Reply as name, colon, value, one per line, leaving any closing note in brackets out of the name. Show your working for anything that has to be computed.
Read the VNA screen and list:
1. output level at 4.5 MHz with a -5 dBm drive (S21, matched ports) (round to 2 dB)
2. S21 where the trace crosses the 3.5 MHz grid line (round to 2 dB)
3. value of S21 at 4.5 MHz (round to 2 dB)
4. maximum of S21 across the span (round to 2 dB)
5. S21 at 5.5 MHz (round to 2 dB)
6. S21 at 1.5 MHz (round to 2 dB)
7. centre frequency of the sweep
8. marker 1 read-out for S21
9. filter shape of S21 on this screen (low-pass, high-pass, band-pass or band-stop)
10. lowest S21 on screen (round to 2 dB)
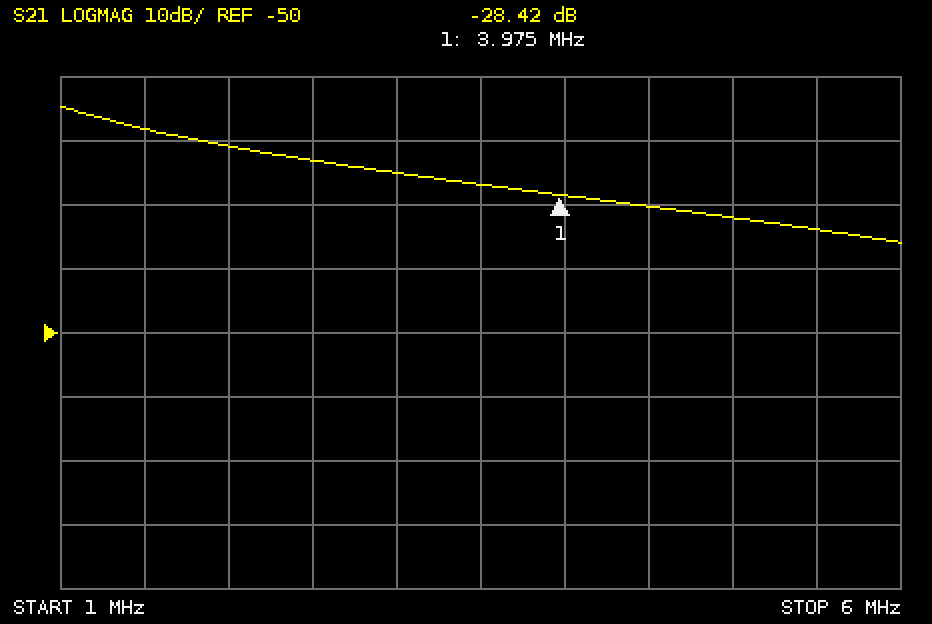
output level at 4.5 MHz with a -5 dBm drive (S21, matched ports): -5 dBm + (-30 dB) = -36 dBm
S21 where the trace crosses the 3.5 MHz grid line: -26 dB
value of S21 at 4.5 MHz: -30 dB
maximum of S21 across the span: -14 dB
S21 at 5.5 MHz: -34 dB
S21 at 1.5 MHz: -18 dB
centre frequency of the sweep: 3.5 MHz
marker 1 read-out for S21: -28.42 dB
filter shape of S21 on this screen: low-pass
lowest S21 on screen: -36 dB
